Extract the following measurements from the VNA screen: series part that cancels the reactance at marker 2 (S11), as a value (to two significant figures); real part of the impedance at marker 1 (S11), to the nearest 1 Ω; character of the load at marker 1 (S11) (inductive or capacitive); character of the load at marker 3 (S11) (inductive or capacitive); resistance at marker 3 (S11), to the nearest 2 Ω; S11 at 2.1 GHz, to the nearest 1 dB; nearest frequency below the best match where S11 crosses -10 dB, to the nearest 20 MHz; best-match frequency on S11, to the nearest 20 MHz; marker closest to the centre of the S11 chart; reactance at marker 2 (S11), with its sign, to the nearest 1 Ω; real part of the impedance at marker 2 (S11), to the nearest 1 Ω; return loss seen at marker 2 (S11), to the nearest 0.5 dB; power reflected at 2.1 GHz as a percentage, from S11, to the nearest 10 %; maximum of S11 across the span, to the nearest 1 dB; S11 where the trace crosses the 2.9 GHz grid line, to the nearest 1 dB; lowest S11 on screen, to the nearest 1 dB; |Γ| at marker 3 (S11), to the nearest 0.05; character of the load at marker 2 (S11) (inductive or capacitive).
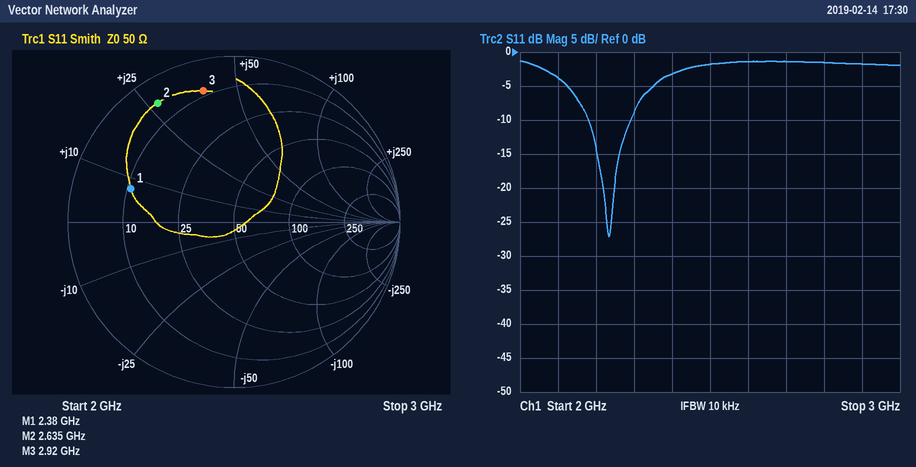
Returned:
2.2 pF
11 Ω
inductive
inductive
8 Ω
-4 dB
2.18 GHz
2.24 GHz
marker 1
+27 Ω
5 Ω
1.5 dB
40 %
-1 dB
-2 dB
-27 dB
0.80
inductive
